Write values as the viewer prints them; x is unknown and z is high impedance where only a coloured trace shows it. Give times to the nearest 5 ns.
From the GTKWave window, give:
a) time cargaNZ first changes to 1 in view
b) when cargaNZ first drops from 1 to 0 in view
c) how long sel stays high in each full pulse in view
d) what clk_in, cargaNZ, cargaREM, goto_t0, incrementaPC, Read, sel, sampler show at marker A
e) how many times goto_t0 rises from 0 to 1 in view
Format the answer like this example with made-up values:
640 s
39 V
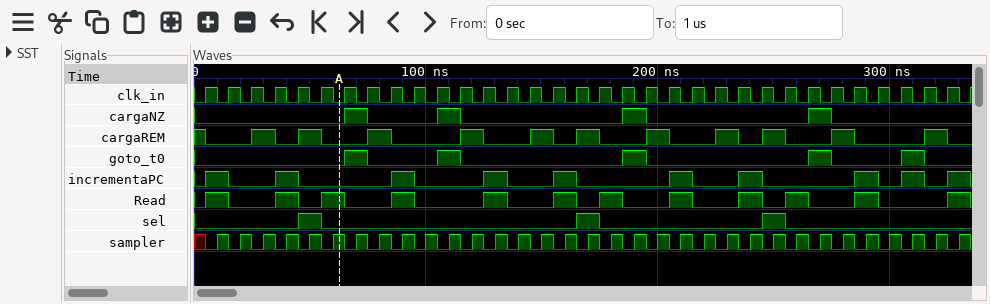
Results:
65 ns
75 ns
10 ns, 10 ns, 10 ns
clk_in=0, cargaNZ=0, cargaREM=0, goto_t0=0, incrementaPC=0, Read=1, sel=0, sampler=1
5
